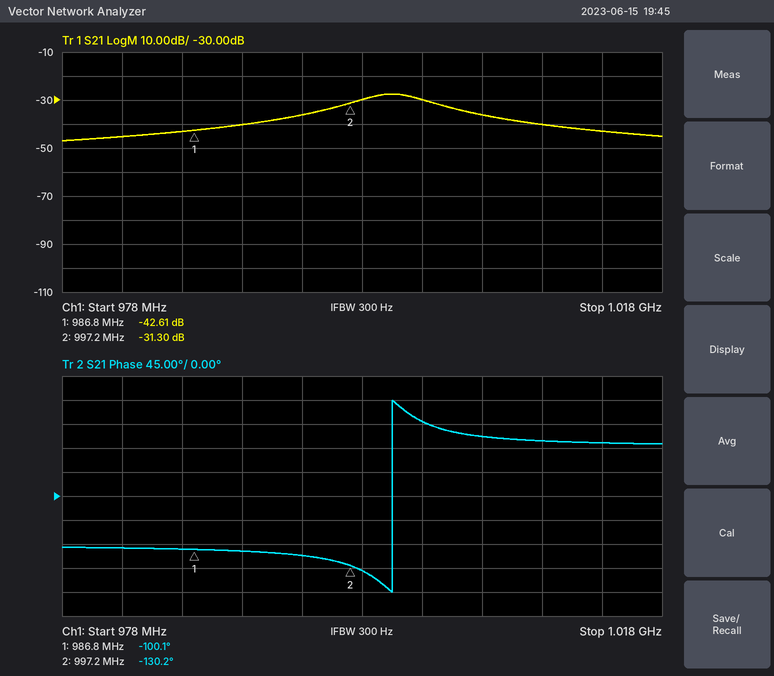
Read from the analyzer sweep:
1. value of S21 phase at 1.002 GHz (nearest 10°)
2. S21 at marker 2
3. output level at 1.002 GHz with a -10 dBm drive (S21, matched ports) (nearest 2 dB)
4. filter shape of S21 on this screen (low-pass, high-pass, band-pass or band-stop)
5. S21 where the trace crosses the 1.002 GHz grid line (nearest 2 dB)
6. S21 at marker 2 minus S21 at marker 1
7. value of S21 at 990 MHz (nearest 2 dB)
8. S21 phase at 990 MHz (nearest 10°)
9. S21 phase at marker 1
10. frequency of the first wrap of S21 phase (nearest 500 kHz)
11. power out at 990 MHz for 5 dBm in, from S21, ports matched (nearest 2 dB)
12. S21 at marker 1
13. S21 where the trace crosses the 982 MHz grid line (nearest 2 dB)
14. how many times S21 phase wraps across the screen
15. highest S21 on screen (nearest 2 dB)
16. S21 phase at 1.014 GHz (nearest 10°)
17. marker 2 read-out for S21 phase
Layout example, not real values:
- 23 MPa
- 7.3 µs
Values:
- 140°
- -31.30 dB
- -40 dBm
- band-pass
- -30 dB
- 11.31 dB
- -40 dB
- -100°
- -100.1°
- 1.0000 GHz
- -36 dBm
- -42.61 dB
- -46 dB
- 1
- -28 dB
- 100°
- -130.2°
